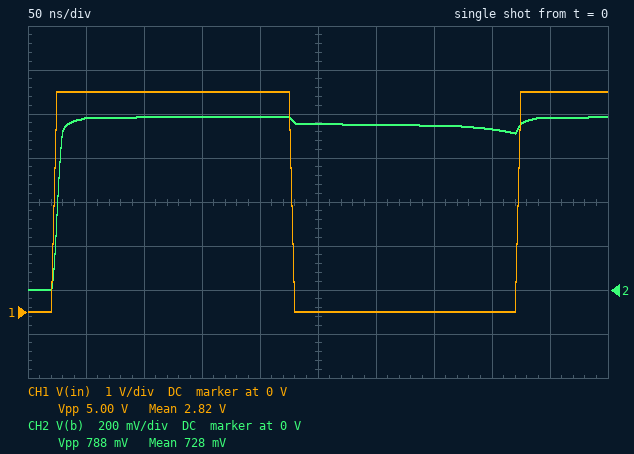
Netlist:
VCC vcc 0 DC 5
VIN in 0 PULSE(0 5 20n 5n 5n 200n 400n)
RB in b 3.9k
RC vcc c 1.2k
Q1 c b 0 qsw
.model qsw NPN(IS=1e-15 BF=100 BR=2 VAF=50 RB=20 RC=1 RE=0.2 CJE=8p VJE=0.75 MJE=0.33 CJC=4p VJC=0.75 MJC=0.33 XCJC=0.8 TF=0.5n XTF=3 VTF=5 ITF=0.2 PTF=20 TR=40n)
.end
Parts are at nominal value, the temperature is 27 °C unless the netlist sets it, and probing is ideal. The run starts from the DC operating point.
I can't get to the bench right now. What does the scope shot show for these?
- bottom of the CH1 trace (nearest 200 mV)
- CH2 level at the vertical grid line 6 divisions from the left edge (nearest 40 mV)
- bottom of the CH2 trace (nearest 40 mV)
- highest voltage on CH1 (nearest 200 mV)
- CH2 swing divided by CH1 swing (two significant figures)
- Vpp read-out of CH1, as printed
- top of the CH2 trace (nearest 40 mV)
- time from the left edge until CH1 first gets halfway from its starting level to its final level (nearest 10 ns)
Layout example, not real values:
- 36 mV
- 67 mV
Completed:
- 0 V
- 760 mV
- 0 V
- 5.0 V
- 0.16
- 5.00 V
- 800 mV
- 20 ns
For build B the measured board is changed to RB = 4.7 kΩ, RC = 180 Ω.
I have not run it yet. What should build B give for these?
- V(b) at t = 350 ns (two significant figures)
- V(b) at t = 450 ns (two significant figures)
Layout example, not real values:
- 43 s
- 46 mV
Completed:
- 770 mV
- 810 mV
